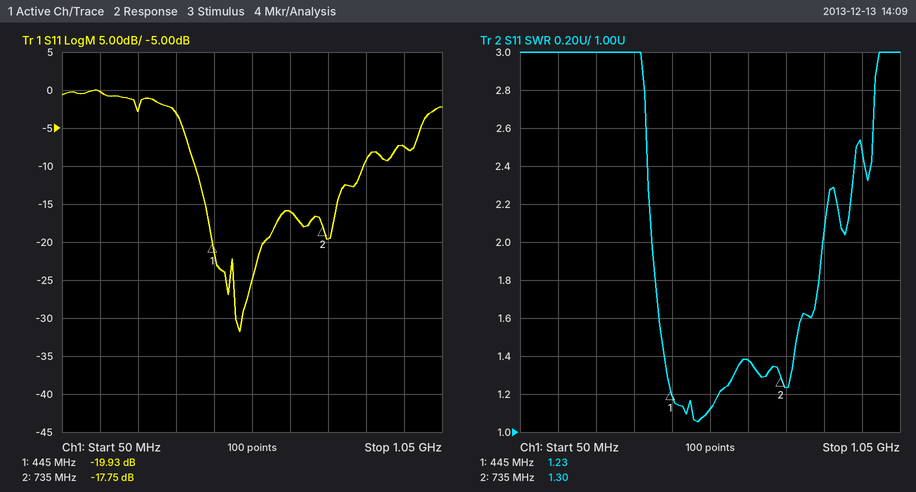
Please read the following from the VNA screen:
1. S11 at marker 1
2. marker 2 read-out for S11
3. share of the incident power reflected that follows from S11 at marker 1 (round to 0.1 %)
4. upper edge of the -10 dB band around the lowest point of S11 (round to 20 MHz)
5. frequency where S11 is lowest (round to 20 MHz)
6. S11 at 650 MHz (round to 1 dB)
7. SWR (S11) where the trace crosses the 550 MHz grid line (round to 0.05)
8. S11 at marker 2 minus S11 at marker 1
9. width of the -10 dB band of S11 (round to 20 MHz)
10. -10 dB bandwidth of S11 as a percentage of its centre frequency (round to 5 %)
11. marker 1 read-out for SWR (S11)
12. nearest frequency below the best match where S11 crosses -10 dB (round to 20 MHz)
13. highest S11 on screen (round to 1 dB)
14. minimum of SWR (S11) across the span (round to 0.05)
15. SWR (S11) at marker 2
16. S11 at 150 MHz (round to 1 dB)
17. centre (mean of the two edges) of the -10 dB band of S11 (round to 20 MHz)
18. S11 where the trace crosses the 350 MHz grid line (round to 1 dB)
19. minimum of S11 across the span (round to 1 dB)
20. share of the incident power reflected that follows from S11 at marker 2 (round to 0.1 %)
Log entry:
-19.93 dB
-17.75 dB
1.0 %
840 MHz
520 MHz
-16 dB
1.10
2.18 dB
440 MHz
70 %
1.23
400 MHz
0 dB
1.05
1.30
0 dB
620 MHz
-3 dB
-32 dB
1.7 %
